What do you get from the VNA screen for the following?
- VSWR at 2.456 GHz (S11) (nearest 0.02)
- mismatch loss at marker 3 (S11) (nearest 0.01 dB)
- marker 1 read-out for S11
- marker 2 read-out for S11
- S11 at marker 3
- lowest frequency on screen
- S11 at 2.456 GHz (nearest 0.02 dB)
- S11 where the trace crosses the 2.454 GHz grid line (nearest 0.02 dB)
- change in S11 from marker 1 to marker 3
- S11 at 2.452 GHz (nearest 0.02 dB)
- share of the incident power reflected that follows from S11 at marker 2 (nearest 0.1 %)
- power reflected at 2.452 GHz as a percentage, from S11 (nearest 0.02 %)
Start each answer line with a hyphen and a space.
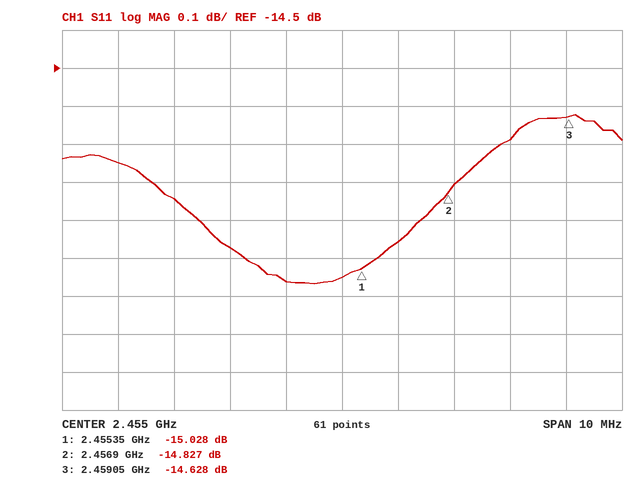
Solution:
- 1.44
- 0.15 dB
- -15.028 dB
- -14.827 dB
- -14.628 dB
- 2.45 GHz
- -14.96 dB
- -15.06 dB
- 0.400 dB
- -14.84 dB
- 3.3 %
- 3.28 %
